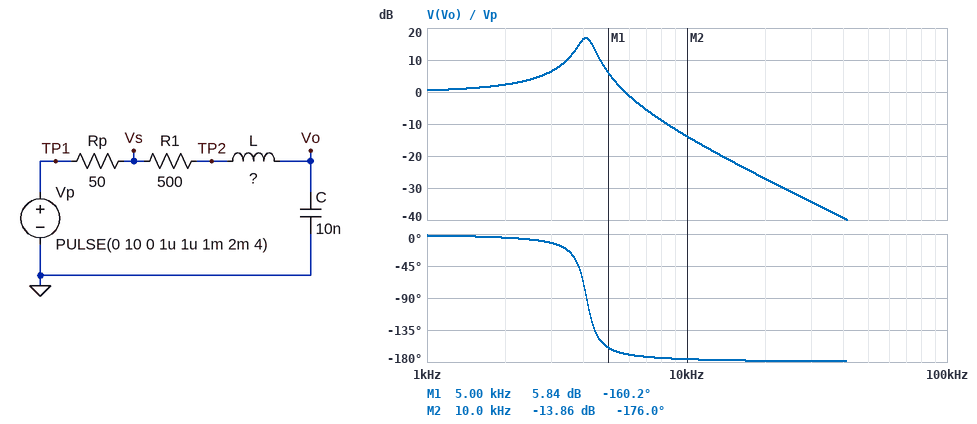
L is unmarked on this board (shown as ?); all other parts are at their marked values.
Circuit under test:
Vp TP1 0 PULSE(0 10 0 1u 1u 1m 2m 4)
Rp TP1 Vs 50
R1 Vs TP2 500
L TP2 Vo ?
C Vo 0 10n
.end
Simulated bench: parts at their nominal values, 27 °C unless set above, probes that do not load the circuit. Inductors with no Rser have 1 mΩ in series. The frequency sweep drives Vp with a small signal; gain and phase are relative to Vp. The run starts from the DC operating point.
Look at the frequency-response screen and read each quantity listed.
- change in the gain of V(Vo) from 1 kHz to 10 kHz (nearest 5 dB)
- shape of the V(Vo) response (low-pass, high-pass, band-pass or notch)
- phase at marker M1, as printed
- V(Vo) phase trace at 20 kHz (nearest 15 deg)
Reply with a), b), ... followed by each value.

a) -15 dB
b) low-pass
c) -160.2 deg
d) -180 deg
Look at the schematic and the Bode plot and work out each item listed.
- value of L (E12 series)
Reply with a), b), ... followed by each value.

a) 150 mH
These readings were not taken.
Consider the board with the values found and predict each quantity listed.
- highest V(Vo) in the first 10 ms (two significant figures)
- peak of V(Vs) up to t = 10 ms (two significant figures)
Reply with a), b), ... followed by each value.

a) 18 V
b) 10 V
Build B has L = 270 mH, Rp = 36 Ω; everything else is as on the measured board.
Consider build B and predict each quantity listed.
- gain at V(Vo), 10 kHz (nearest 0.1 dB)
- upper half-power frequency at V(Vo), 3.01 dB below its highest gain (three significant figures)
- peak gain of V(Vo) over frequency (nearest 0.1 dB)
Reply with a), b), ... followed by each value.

a) -19.7 dB
b) 3.21 kHz
c) 19.7 dB
